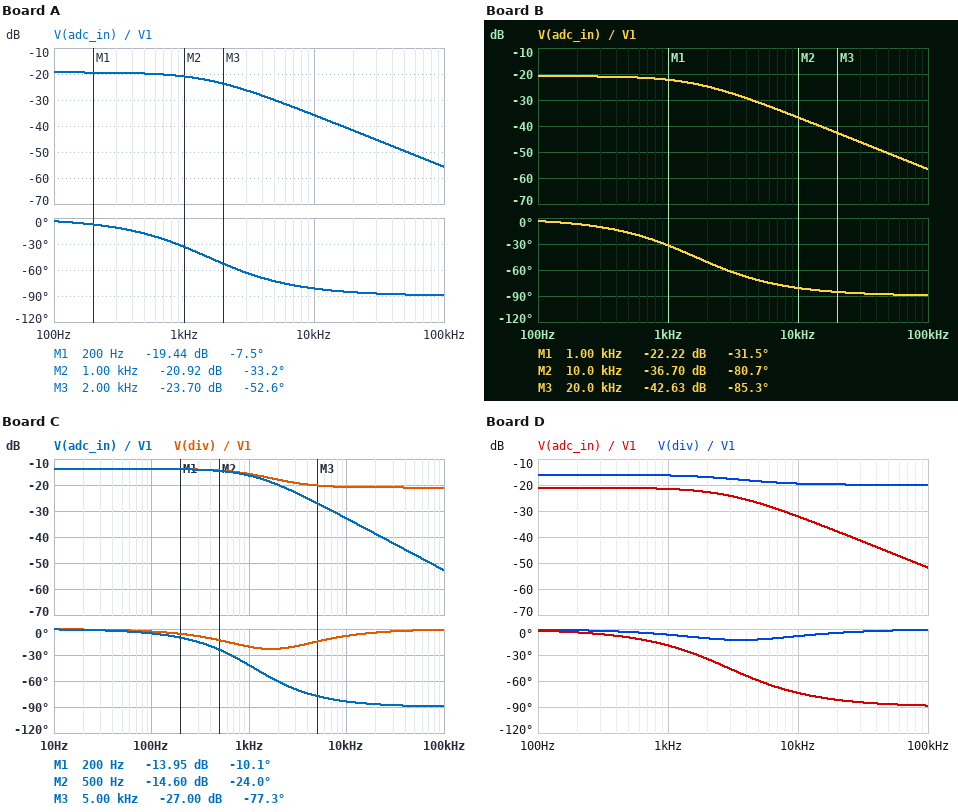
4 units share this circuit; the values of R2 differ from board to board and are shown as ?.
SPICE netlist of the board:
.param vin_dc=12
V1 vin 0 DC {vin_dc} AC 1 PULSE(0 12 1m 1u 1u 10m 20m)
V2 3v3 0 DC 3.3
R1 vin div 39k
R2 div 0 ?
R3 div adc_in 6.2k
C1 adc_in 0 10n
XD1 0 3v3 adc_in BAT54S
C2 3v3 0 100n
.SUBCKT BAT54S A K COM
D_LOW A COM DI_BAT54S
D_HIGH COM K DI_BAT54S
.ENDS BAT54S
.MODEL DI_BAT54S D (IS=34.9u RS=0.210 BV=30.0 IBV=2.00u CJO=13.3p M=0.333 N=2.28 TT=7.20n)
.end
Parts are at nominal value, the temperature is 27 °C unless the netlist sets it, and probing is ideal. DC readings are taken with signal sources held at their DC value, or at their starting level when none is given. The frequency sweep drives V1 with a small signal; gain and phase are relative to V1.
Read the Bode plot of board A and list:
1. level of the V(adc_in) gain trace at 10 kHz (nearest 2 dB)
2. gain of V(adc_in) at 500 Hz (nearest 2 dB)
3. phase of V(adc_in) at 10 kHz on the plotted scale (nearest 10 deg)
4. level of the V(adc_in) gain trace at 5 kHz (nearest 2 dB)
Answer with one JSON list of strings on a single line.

["-36 dB", "-20 dB", "-80 deg", "-30 dB"]
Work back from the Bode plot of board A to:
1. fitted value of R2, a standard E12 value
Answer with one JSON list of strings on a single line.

["4.7 kΩ"]
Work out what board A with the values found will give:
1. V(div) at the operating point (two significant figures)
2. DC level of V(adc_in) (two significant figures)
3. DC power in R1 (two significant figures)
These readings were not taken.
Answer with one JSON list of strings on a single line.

["1.3 V", "1.3 V", "2.9 mW"]
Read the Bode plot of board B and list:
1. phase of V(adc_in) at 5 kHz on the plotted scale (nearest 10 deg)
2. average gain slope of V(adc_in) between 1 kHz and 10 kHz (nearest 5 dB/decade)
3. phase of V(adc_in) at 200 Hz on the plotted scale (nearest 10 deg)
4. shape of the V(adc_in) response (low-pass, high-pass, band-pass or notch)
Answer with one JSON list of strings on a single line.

["-70 deg", "-15 dB/decade", "-10 deg", "low-pass"]
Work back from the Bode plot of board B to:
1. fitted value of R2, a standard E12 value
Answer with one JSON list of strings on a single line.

["3.9 kΩ"]
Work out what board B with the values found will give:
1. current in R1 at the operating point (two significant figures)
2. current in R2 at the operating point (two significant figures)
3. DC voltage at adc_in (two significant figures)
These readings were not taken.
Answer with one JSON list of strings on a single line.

["280 µA", "280 µA", "1.1 V"]
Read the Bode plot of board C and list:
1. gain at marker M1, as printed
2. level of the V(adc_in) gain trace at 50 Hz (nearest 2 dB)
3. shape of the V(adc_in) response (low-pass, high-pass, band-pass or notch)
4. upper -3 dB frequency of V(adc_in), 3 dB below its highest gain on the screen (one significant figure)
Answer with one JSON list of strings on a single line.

["-13.95 dB", "-14 dB", "low-pass", "1 kHz"]
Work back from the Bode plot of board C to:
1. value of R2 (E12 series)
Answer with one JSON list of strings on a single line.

["10 kΩ"]
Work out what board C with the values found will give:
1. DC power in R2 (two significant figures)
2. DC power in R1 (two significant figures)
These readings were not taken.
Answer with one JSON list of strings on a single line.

["600 µW", "2.3 mW"]
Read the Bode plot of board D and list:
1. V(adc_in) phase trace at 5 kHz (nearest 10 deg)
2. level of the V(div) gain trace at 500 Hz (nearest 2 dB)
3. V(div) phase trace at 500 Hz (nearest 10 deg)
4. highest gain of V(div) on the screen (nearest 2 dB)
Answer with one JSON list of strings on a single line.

["-60 deg", "-16 dB", "0 deg", "-16 dB"]
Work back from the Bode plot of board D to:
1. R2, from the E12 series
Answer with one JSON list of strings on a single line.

["15 kΩ"]
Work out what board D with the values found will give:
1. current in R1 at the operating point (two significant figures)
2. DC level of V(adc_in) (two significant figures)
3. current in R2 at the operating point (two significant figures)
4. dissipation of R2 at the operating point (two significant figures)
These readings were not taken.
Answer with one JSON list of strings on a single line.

["220 µA", "3.2 V", "220 µA", "710 µW"]
